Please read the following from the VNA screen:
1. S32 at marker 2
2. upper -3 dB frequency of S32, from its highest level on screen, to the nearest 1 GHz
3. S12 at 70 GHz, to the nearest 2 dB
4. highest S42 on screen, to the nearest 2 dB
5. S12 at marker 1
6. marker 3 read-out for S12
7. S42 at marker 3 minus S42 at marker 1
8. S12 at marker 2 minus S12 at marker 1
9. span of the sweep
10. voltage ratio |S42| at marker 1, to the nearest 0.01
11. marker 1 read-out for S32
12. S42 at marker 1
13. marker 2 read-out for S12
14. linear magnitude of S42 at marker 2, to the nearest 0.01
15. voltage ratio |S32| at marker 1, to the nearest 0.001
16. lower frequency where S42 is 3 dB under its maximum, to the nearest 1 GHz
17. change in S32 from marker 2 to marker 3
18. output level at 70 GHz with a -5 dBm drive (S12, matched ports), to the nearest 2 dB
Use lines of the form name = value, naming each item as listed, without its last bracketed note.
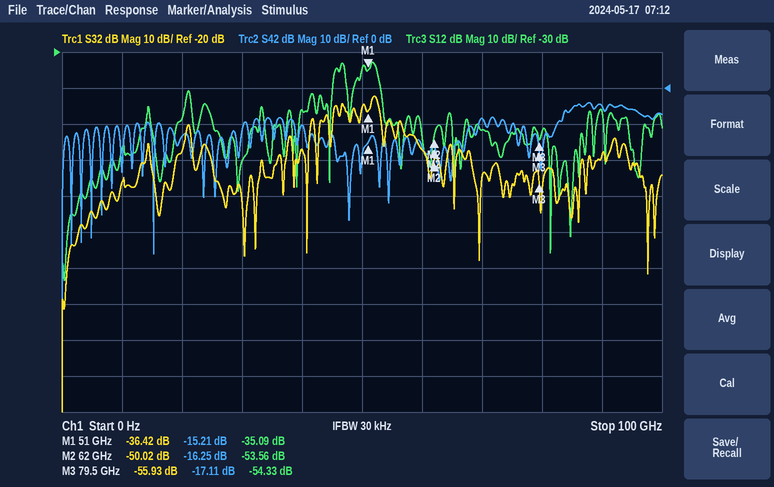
S32 at marker 2 = -50.02 dB
upper -3 dB frequency of S32, from its highest level on screen, to the nearest 1 GHz = 53 GHz
S12 at 70 GHz, to the nearest 2 dB = -52 dB
highest S42 on screen, to the nearest 2 dB = -4 dB
S12 at marker 1 = -35.09 dB
marker 3 read-out for S12 = -54.33 dB
S42 at marker 3 minus S42 at marker 1 = -1.90 dB
S12 at marker 2 minus S12 at marker 1 = -18.47 dB
span of the sweep = 100 GHz
voltage ratio |S42| at marker 1, to the nearest 0.01 = 0.17
marker 1 read-out for S32 = -36.42 dB
S42 at marker 1 = -15.21 dB
marker 2 read-out for S12 = -53.56 dB
linear magnitude of S42 at marker 2, to the nearest 0.01 = 0.15
voltage ratio |S32| at marker 1, to the nearest 0.001 = 0.015
lower frequency where S42 is 3 dB under its maximum, to the nearest 1 GHz = 84 GHz
change in S32 from marker 2 to marker 3 = -5.91 dB
output level at 70 GHz with a -5 dBm drive (S12, matched ports), to the nearest 2 dB = -56 dBm
